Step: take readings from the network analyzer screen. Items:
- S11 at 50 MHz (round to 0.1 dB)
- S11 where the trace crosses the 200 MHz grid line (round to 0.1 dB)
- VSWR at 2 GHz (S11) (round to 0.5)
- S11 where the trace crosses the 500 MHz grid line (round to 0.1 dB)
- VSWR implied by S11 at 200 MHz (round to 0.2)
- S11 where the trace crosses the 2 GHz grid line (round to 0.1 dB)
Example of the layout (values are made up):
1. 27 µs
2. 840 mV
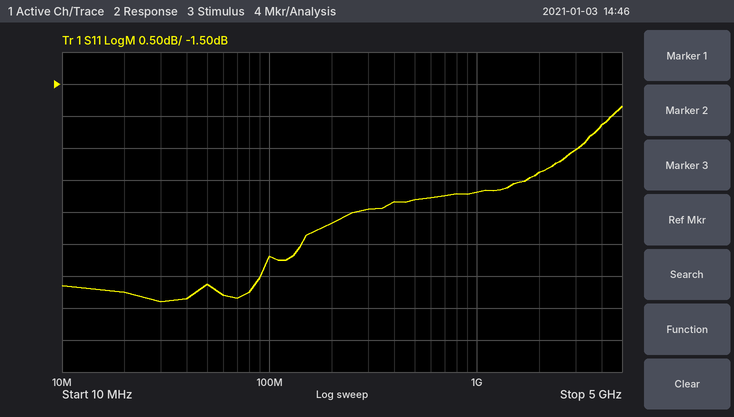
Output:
1. -4.6 dB
2. -3.7 dB
3. 6.0
4. -3.3 dB
5. 4.8
6. -2.9 dB
